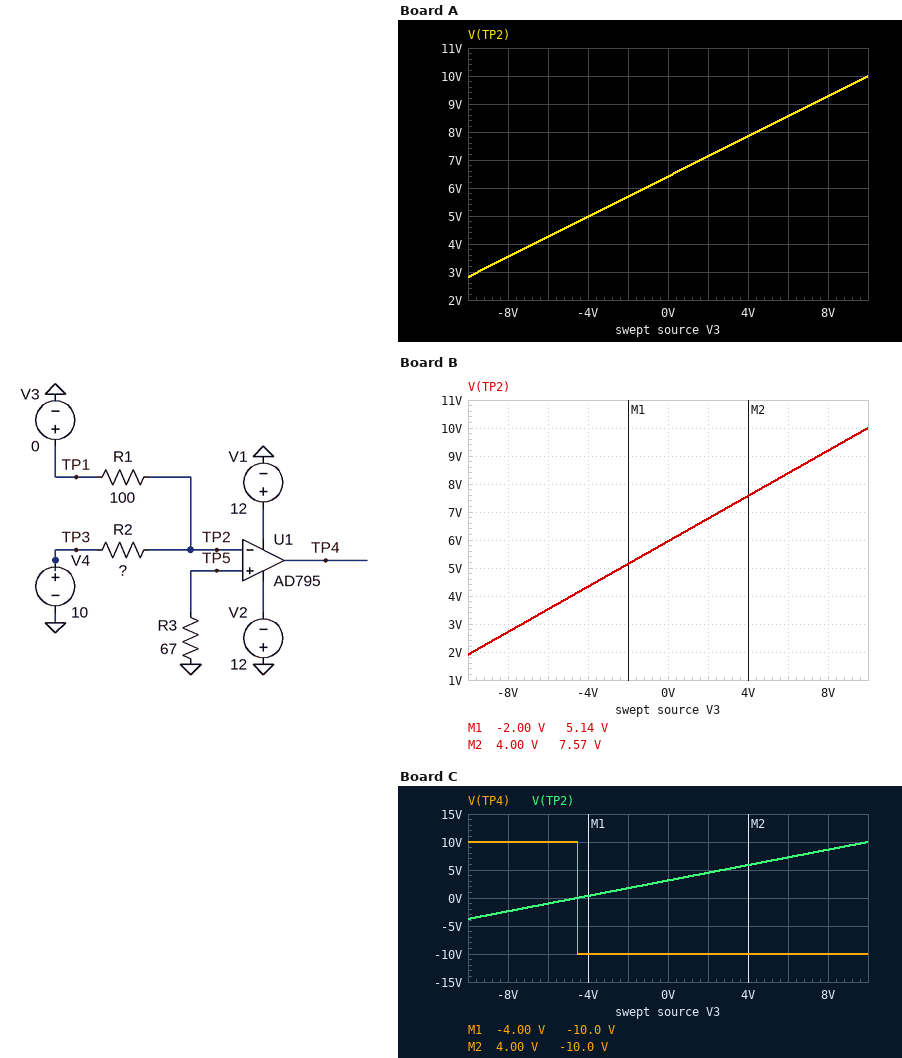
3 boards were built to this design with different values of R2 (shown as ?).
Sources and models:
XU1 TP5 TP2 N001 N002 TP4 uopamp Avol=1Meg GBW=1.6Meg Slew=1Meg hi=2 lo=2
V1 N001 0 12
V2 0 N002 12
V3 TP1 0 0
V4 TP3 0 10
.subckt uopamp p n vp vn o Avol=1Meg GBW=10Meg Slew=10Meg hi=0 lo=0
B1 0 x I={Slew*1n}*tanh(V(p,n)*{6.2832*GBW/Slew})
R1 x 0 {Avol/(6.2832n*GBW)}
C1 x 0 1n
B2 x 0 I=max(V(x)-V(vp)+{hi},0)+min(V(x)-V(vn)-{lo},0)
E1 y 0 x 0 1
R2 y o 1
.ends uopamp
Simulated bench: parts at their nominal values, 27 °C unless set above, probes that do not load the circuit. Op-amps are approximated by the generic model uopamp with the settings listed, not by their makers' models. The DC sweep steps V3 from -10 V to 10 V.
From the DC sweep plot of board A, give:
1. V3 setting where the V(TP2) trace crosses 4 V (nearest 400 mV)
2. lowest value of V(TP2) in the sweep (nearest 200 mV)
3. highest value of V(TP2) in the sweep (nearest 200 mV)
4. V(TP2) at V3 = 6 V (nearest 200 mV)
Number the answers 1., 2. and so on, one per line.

1. -6.8 V
2. 2.8 V
3. 10.0 V
4. 8.6 V
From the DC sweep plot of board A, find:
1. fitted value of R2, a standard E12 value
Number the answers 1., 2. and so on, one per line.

1. 56 Ω
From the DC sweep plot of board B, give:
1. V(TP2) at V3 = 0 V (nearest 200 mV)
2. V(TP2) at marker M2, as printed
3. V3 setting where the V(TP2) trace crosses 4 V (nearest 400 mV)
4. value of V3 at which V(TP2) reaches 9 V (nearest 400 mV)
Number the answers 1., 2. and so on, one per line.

1. 6.0 V
2. 7.57 V
3. -4.8 V
4. 7.6 V
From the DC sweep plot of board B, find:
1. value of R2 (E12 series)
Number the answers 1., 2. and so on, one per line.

1. 68 Ω
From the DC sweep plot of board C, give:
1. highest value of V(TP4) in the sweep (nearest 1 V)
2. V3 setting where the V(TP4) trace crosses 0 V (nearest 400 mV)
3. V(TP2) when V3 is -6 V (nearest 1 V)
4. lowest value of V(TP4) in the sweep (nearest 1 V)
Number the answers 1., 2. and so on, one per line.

1. 10 V
2. -4.4 V
3. -1 V
4. -10 V
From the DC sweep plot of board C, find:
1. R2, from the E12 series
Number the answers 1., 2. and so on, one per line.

1. 220 Ω
